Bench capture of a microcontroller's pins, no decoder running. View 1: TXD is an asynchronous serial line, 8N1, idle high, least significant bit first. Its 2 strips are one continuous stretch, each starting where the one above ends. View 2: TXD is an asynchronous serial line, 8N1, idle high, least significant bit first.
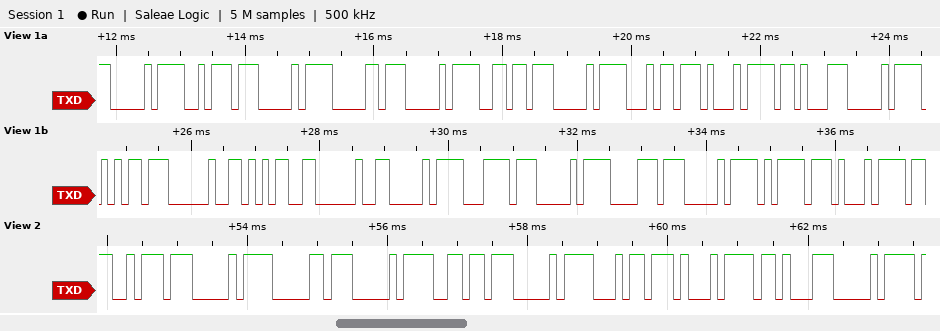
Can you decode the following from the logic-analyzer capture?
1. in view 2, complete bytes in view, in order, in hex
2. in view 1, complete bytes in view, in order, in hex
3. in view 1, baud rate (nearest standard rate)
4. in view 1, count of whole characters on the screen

BA D0 B0 D0 B6 D0 B4 D1 8B D0
D0 BA D0 B0 D0 B6 D0 B4 D1 8B D0 B5 20 35 20 D0 BC D0 B8 D0 BD D1
9600 baud
22
